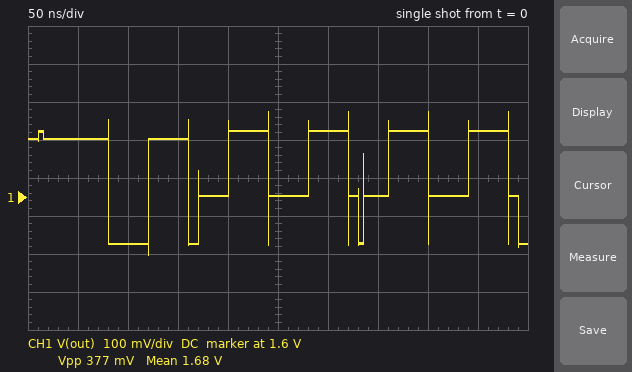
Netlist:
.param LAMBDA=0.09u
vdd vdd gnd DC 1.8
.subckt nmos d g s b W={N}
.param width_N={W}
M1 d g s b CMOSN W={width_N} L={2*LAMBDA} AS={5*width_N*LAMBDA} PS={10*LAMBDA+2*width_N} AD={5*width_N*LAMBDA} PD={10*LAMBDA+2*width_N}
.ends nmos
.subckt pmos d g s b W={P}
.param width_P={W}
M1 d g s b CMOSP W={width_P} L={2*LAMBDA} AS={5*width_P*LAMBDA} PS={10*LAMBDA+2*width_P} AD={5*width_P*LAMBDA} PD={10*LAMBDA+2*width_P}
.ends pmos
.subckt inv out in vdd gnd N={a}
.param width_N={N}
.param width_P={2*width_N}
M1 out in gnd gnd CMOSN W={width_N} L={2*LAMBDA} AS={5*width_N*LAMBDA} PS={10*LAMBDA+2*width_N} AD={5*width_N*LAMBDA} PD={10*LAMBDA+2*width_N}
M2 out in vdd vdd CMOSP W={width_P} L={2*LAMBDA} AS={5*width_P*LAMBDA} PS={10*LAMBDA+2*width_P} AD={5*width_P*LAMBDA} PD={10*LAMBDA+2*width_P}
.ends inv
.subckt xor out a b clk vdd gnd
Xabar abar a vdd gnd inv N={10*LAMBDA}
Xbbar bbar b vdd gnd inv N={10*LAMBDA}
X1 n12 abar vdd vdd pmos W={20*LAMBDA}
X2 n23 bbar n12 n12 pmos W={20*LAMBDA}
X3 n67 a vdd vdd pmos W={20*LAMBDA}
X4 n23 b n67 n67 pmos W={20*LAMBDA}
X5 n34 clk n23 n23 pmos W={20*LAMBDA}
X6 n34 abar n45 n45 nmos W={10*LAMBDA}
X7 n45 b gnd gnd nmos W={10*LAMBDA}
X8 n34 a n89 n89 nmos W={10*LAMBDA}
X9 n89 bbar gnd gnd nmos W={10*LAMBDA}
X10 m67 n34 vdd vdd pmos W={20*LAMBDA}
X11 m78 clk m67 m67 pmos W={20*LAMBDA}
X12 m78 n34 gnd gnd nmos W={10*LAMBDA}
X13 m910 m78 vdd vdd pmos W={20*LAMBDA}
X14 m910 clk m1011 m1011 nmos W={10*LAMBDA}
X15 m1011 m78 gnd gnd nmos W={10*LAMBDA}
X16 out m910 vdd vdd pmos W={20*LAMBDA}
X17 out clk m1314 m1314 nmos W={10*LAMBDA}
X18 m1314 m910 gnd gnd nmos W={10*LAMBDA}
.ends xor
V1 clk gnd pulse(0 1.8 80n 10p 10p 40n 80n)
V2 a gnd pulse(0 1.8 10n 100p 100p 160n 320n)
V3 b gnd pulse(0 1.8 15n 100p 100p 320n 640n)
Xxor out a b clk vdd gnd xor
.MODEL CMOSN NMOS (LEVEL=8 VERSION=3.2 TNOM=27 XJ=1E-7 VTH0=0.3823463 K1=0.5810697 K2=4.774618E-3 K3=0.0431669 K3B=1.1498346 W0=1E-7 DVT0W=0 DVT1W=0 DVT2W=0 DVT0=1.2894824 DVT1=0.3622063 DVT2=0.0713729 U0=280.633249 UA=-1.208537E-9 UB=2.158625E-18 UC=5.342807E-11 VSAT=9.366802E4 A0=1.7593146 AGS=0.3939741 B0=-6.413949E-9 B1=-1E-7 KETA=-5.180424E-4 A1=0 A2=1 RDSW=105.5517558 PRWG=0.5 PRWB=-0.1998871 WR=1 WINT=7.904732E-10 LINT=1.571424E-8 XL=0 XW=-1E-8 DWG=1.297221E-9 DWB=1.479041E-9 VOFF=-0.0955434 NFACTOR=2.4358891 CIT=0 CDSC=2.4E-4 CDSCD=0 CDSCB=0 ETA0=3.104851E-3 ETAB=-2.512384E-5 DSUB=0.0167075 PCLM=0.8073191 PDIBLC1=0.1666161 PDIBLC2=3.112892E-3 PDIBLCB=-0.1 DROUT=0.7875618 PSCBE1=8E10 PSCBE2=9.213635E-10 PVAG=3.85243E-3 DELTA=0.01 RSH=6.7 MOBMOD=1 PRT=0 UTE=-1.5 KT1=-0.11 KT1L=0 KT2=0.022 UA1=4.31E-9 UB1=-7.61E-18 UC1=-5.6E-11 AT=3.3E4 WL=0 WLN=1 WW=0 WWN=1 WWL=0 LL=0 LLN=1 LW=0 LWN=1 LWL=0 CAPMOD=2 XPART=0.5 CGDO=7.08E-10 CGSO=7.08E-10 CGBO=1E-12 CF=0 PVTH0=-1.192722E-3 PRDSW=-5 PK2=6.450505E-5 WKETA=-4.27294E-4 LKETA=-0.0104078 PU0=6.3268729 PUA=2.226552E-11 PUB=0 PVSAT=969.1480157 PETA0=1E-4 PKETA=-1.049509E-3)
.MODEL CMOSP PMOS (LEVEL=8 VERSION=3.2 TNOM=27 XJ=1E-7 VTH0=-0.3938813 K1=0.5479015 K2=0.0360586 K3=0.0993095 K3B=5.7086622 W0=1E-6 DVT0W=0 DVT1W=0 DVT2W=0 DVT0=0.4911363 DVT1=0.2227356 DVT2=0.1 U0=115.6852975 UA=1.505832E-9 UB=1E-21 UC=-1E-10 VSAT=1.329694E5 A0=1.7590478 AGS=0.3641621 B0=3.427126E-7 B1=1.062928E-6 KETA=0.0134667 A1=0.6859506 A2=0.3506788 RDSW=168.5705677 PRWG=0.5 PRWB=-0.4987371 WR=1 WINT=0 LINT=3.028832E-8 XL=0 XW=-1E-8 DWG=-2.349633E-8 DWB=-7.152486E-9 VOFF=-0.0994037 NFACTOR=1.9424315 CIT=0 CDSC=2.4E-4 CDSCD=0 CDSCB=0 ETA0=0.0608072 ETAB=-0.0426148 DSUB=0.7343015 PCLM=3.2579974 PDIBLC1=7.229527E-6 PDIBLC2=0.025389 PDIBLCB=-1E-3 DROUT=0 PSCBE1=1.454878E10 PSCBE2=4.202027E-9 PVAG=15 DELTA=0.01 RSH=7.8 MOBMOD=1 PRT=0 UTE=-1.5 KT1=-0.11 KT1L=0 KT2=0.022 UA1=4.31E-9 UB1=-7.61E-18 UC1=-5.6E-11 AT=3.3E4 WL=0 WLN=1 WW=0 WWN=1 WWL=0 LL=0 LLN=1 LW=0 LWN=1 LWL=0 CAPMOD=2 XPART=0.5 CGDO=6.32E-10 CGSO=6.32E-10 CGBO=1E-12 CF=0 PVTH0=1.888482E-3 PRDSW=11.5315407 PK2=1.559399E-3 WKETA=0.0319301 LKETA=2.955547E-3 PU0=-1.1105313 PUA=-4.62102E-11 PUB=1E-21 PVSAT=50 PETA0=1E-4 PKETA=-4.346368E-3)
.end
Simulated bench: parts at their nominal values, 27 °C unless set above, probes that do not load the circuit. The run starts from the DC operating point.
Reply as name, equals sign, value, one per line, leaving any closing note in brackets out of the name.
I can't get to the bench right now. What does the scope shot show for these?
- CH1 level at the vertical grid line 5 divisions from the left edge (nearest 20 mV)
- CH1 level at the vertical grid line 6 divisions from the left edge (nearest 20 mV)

CH1 level at the vertical grid line 5 divisions from the left edge = 1.60 V
CH1 level at the vertical grid line 6 divisions from the left edge = 1.78 V
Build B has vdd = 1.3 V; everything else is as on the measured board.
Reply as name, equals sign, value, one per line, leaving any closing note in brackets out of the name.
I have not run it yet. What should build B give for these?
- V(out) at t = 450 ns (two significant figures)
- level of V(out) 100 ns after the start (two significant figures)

V(out) at t = 450 ns = 1.3 V
level of V(out) 100 ns after the start = 1.1 V
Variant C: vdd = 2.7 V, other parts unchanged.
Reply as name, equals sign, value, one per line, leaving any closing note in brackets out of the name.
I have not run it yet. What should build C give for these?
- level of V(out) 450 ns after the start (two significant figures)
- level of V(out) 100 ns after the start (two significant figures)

level of V(out) 450 ns after the start = 2.6 V
level of V(out) 100 ns after the start = 2.3 V
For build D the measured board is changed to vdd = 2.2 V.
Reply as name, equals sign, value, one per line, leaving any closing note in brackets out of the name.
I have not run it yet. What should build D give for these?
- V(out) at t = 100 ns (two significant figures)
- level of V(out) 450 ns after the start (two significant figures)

V(out) at t = 100 ns = 1.8 V
level of V(out) 450 ns after the start = 2.1 V
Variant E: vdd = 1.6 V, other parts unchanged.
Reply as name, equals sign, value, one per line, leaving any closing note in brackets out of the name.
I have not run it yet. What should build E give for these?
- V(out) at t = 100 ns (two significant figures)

V(out) at t = 100 ns = 1.3 V
